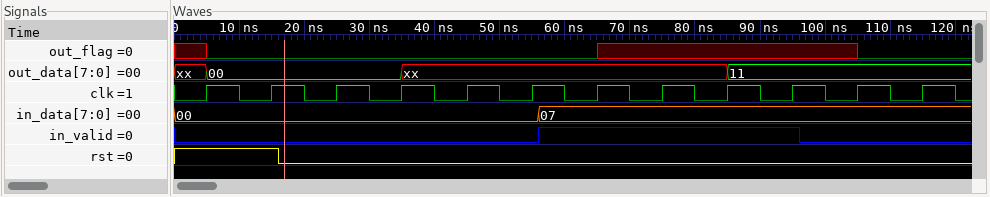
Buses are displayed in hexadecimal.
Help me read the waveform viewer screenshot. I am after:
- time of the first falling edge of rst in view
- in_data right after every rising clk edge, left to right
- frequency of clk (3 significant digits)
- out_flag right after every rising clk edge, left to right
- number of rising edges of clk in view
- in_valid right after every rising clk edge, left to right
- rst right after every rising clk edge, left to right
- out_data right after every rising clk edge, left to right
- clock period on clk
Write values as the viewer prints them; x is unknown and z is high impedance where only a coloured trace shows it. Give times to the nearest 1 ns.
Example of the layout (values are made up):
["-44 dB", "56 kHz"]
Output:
["16 ns", "00, 00, 00, 00, 00, 00, 07, 07, 07, 07, 07, 07", "100 MHz", "0 0 0 0 0 0 x x x x 0 0", "12", "0 0 0 0 0 0 1 1 1 1 0 0", "1 1 0 0 0 0 0 0 0 0 0 0", "00, 00, 00, xx, xx, xx, xx, xx, 11, 11, 11, 11", "10 ns"]
